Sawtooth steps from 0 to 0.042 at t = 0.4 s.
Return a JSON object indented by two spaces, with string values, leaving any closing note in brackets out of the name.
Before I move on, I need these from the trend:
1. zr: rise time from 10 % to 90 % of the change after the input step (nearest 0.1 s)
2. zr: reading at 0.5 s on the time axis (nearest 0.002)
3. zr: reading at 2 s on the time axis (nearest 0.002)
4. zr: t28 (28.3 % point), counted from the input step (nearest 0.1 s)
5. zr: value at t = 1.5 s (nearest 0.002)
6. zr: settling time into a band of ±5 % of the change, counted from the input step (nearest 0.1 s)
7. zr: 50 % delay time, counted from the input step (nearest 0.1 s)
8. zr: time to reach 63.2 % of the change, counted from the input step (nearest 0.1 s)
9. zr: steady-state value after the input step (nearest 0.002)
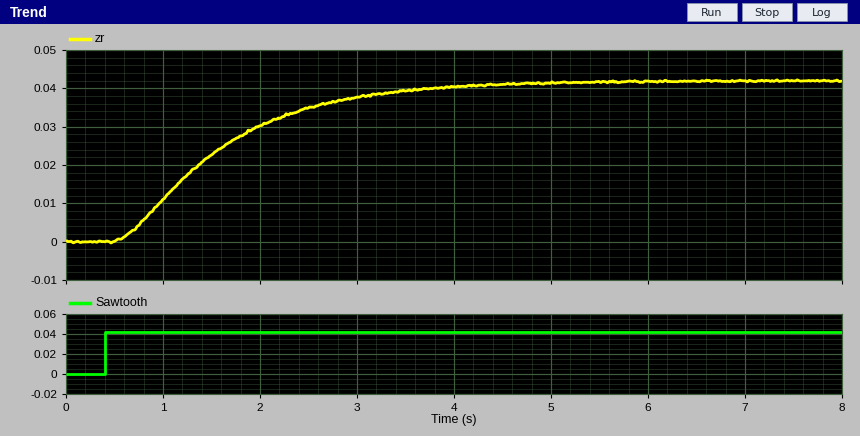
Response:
{
  "zr: rise time from 10 % to 90 % of the change after the input step": "2.3 s",
  "zr: reading at 0.5 s on the time axis": "0.000",
  "zr: reading at 2 s on the time axis": "0.030",
  "zr: t28 (28.3 % point), counted from the input step": "0.6 s",
  "zr: value at t = 1.5 s": "0.022",
  "zr: settling time into a band of ±5 % of the change, counted from the input step": "3.3 s",
  "zr: 50 % delay time, counted from the input step": "1.0 s",
  "zr: time to reach 63.2 % of the change, counted from the input step": "1.3 s",
  "zr: steady-state value after the input step": "0.042"
}
